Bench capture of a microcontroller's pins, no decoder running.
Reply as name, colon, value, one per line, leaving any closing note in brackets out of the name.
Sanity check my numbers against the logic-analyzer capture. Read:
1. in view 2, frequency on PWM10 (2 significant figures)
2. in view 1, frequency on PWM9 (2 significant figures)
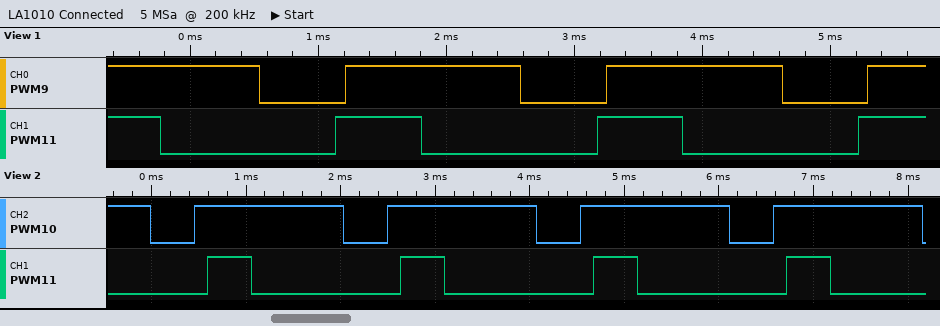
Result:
in view 2, frequency on PWM10: 490 Hz
in view 1, frequency on PWM9: 490 Hz
